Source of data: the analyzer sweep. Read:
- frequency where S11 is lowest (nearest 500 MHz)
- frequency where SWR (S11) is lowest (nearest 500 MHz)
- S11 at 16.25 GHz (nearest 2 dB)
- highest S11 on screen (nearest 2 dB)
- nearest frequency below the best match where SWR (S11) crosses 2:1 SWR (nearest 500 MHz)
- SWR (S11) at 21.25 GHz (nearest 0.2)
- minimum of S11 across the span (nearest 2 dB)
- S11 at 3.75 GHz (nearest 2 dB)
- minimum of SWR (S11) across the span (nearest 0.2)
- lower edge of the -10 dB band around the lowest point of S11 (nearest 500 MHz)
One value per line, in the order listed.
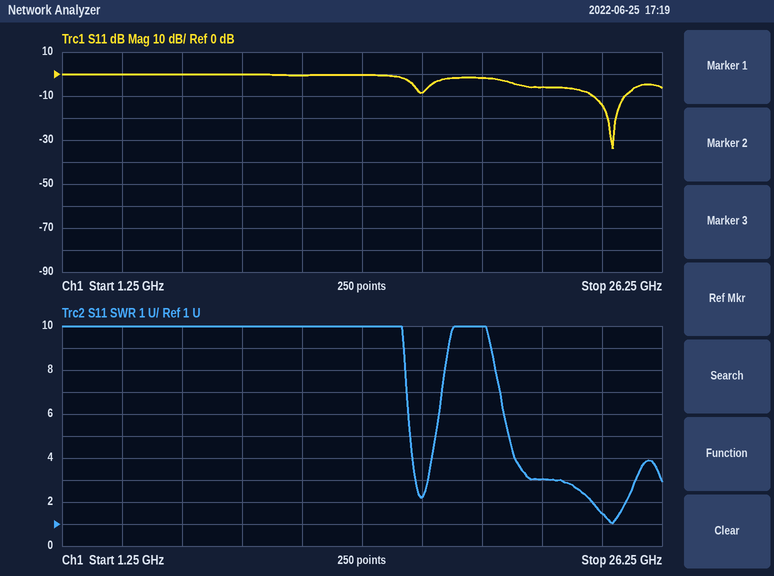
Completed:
24.0 GHz
24.0 GHz
-8 dB
0 dB
23.5 GHz
3.0
-34 dB
0 dB
1.0
23.5 GHz
